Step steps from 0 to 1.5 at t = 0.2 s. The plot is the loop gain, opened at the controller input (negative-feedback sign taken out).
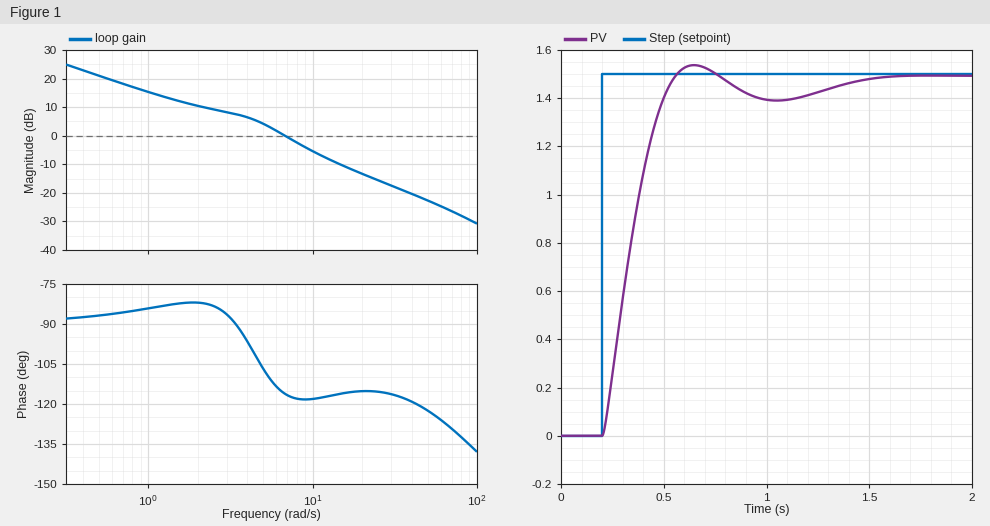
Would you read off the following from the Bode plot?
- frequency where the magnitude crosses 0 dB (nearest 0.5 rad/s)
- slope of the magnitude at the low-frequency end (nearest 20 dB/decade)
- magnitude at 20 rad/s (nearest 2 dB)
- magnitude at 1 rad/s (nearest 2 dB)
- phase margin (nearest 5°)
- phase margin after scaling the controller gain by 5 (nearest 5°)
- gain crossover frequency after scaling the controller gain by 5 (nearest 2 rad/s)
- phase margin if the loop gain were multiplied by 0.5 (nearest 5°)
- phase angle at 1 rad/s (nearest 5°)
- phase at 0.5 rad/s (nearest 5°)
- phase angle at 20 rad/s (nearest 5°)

7.0 rad/s
-20 dB/decade
-14 dB
16 dB
65°
65°
22 rad/s
80°
-85°
-85°
-115°
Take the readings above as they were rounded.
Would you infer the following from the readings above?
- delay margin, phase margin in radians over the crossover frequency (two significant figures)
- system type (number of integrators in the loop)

0.16 s
1
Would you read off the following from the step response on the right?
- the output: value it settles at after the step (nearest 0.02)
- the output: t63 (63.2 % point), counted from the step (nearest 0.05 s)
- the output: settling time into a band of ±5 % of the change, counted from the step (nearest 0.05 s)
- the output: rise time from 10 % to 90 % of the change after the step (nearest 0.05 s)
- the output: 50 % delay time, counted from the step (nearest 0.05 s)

1.50
0.15 s
1.05 s
0.25 s
0.15 s
